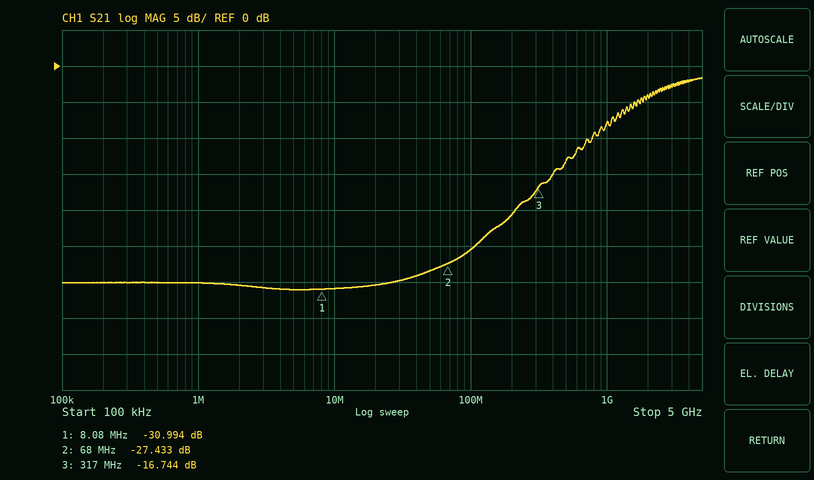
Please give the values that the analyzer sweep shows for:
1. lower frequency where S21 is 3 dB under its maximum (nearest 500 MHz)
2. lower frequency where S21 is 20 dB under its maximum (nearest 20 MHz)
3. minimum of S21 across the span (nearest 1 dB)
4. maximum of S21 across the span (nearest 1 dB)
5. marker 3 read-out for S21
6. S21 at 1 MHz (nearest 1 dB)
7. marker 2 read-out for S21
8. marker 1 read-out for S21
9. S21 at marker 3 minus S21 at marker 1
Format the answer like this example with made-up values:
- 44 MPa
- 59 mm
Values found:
- 2.0 GHz
- 180 MHz
- -31 dB
- -2 dB
- -16.744 dB
- -30 dB
- -27.433 dB
- -30.994 dB
- 14.250 dB
